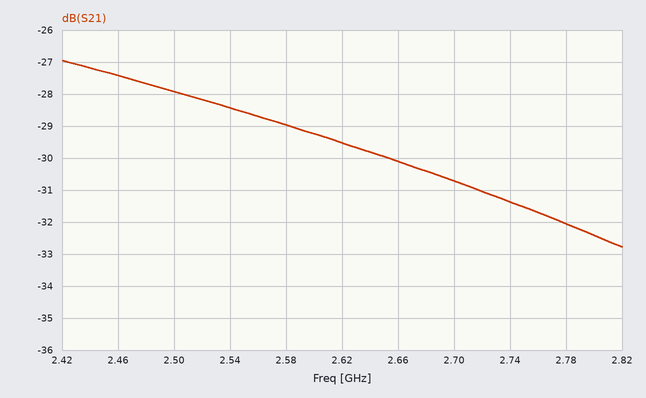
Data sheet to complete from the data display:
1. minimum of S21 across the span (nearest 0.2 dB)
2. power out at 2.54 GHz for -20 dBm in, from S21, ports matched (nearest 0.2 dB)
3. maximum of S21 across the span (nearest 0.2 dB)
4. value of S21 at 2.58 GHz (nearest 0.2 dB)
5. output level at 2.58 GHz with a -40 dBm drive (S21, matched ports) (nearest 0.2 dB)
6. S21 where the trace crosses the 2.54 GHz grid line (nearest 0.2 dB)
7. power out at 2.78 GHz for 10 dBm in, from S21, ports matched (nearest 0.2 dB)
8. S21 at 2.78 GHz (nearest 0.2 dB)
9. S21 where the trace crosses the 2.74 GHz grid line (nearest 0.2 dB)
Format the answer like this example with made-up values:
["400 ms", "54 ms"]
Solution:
["-32.8 dB", "-48.4 dBm", "-27.0 dB", "-29.0 dB", "-69.0 dBm", "-28.4 dB", "-22.0 dBm", "-32.0 dB", "-31.4 dB"]
